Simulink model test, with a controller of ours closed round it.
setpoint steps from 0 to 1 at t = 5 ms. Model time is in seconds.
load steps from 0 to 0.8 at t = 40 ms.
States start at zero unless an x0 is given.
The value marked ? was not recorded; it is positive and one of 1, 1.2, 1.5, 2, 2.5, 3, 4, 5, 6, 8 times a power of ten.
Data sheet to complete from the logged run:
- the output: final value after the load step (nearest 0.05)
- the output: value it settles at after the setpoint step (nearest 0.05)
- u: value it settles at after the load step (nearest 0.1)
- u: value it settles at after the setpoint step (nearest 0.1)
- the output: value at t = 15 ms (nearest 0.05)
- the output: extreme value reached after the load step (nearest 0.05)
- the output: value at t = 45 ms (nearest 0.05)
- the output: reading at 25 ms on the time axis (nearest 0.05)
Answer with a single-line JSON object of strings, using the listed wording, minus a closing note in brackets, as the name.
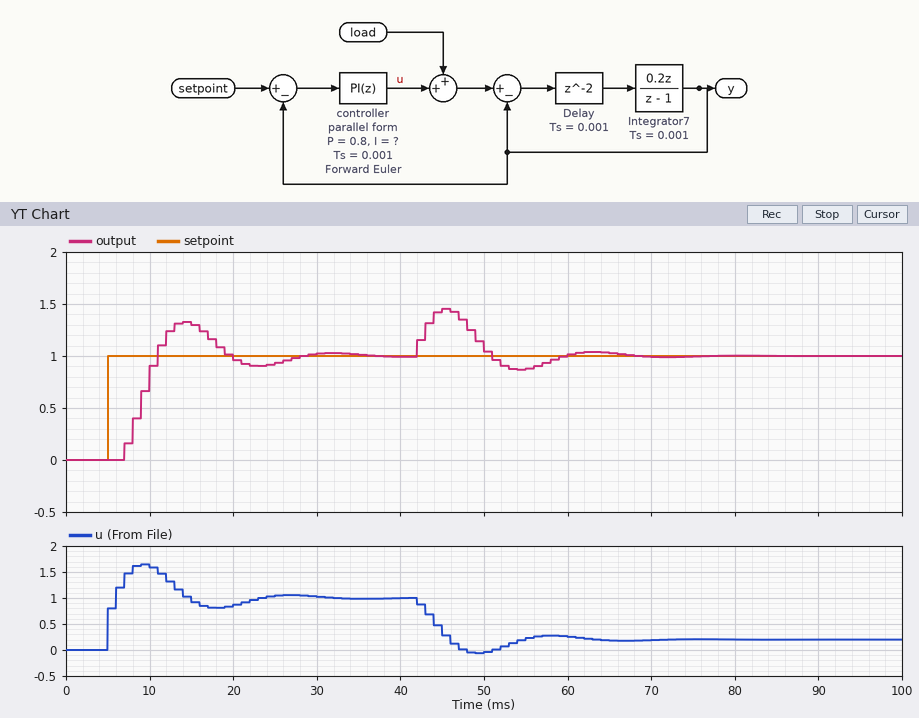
{"the output: final value after the load step": "1.00", "the output: value it settles at after the setpoint step": "1.00", "u: value it settles at after the load step": "0.2", "u: value it settles at after the setpoint step": "1.0", "the output: value at t = 15 ms": "1.30", "the output: extreme value reached after the load step": "1.45", "the output: value at t = 45 ms": "1.45", "the output: reading at 25 ms on the time axis": "0.95"}
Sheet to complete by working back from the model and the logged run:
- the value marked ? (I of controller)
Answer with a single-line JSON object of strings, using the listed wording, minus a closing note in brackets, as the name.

{"the value marked ?": "400"}
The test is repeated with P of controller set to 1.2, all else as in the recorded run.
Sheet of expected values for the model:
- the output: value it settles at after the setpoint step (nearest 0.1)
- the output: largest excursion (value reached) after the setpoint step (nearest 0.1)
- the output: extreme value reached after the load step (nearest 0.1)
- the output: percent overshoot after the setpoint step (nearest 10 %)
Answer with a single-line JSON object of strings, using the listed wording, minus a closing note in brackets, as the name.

{"the output: value it settles at after the setpoint step": "1.0", "the output: largest excursion (value reached) after the setpoint step": "1.2", "the output: extreme value reached after the load step": "1.4", "the output: percent overshoot after the setpoint step": "20 %"}
